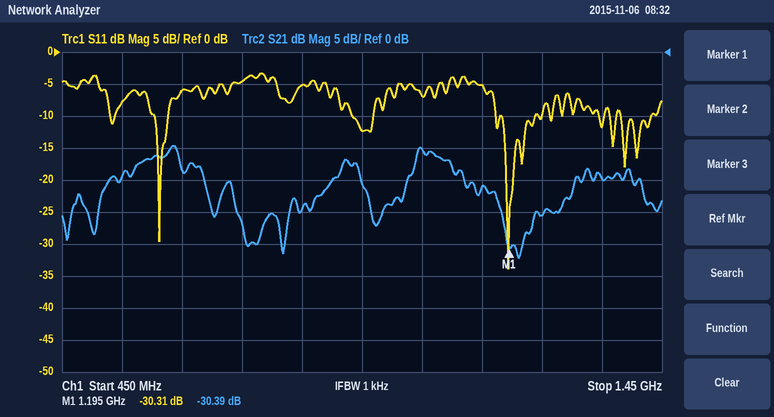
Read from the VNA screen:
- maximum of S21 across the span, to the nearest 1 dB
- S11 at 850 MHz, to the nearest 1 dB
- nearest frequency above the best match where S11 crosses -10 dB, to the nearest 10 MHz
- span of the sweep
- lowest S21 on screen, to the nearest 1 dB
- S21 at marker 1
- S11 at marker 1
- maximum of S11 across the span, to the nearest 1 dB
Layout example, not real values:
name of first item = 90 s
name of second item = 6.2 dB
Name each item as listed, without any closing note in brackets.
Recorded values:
maximum of S21 across the span, to the nearest 1 dB = -15 dB
S11 at 850 MHz, to the nearest 1 dB = -5 dB
nearest frequency above the best match where S11 crosses -10 dB, to the nearest 10 MHz = 1.24 GHz
span of the sweep = 1 GHz
lowest S21 on screen, to the nearest 1 dB = -32 dB
S21 at marker 1 = -30.39 dB
S11 at marker 1 = -30.31 dB
maximum of S11 across the span, to the nearest 1 dB = -3 dB
